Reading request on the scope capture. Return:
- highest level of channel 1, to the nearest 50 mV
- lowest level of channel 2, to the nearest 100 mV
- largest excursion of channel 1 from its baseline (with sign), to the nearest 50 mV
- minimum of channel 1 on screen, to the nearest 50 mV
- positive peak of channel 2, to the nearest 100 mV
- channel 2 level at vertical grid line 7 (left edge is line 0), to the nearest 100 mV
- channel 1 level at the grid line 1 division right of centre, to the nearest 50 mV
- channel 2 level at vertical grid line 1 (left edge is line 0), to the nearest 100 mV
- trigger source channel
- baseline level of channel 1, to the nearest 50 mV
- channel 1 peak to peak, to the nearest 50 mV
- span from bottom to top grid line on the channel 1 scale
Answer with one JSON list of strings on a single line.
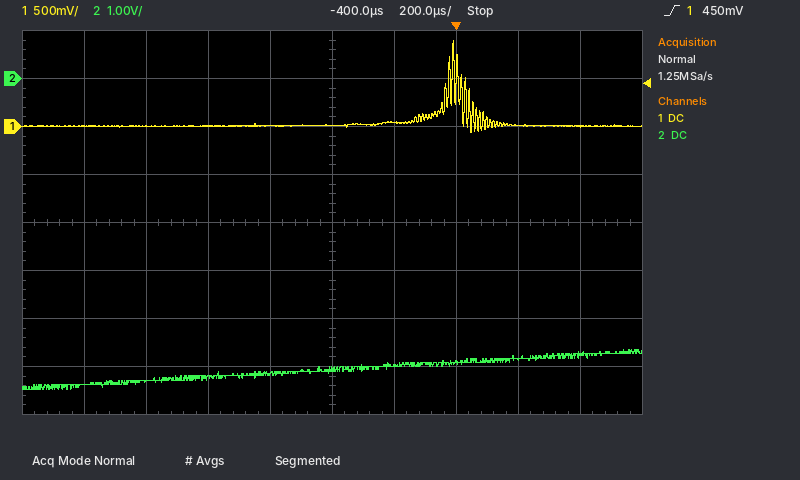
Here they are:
["900 mV", "-6.5 V", "+900 mV", "-50 mV", "-5.6 V", "-5.9 V", "50 mV", "-6.4 V", "channel 1", "0 mV", "950 mV", "4 V"]
